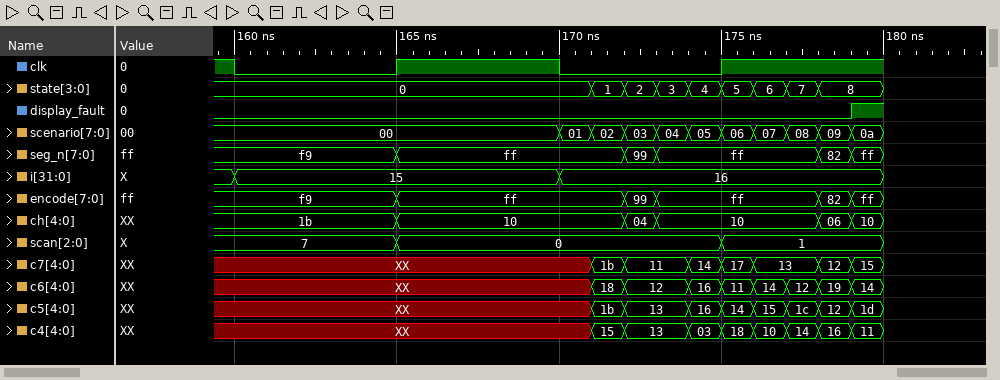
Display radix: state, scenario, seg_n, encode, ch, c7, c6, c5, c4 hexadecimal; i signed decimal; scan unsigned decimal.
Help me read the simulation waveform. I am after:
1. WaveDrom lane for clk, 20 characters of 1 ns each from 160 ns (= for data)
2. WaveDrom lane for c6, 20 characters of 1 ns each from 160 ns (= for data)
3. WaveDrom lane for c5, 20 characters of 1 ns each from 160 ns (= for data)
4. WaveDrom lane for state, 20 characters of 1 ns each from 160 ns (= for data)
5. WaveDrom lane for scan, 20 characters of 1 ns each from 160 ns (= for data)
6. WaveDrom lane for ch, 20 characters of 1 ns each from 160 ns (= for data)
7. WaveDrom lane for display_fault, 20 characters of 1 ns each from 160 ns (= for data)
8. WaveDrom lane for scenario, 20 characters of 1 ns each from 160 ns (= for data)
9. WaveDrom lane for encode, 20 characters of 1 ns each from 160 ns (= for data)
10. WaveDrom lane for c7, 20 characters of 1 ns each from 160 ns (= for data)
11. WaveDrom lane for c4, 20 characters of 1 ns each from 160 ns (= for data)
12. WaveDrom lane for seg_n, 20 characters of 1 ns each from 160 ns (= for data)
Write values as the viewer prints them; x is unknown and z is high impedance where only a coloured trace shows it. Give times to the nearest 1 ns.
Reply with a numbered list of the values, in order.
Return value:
1. {name: 'clk', wave: '0....1....0....1....'}
2. {name: 'c6', wave: 'x..........==.======', data: '18 12 16 11 14 12 19 14'}
3. {name: 'c5', wave: 'x..........==.======', data: '1b 13 16 14 15 1c 12 1d'}
4. {name: 'state', wave: '=..........========.', data: '0 1 2 3 4 5 6 7 8'}
5. {name: 'scan', wave: '=....=.........=....', data: '7 0 1'}
6. {name: 'ch', wave: '=....=......==....==', data: '1b 10 04 10 06 10'}
7. {name: 'display_fault', wave: '0..................1'}
8. {name: 'scenario', wave: '=.........==========', data: '00 01 02 03 04 05 06 07 08 09 0a'}
9. {name: 'encode', wave: '=....=......==....==', data: 'f9 ff 99 ff 82 ff'}
10. {name: 'c7', wave: 'x..........==.===.==', data: '1b 11 14 17 13 12 15'}
11. {name: 'c4', wave: 'x..........==.======', data: '15 13 03 18 10 14 16 11'}
12. {name: 'seg_n', wave: '=....=......==....==', data: 'f9 ff 99 ff 82 ff'}
